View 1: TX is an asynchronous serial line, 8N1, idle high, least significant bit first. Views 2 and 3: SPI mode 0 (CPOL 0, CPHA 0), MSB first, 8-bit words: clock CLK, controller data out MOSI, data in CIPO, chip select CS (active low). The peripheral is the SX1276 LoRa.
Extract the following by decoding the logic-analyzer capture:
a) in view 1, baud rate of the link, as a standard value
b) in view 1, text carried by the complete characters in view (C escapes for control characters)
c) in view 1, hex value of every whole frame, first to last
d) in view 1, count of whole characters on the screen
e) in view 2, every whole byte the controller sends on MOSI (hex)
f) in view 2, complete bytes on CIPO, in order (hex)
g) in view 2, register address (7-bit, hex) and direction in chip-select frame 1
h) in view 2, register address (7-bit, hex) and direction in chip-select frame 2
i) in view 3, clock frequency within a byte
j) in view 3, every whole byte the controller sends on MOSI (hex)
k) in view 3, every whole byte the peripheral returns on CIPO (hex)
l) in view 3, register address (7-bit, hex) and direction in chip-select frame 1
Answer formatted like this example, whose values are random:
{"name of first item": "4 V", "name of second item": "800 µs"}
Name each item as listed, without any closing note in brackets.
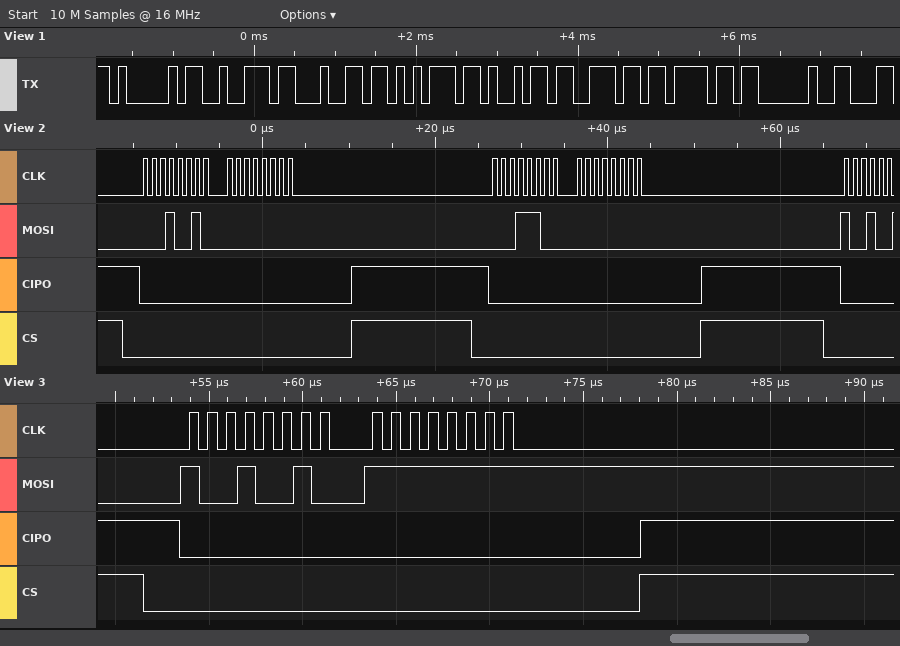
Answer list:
{"in view 1, baud rate of the link, as a standard value": "9600 baud", "in view 1, text carried by the complete characters in view": "\"Arduino \"", "in view 1, hex value of every whole frame, first to last": "41 72 64 75 69 6E 6F 20", "in view 1, count of whole characters on the screen": "8", "in view 2, every whole byte the controller sends on MOSI": "0x12 0x00 0x1C 0x00", "in view 2, complete bytes on CIPO, in order": "0x00 0x00 0x00 0x00", "in view 2, register address (7-bit, hex) and direction in chip-select frame 1": "0x12 read", "in view 2, register address (7-bit, hex) and direction in chip-select frame 2": "0x1C read", "in view 3, clock frequency within a byte": "1 MHz", "in view 3, every whole byte the controller sends on MOSI": "92 FF", "in view 3, every whole byte the peripheral returns on CIPO": "00 00", "in view 3, register address (7-bit, hex) and direction in chip-select frame 1": "0x12 write"}
